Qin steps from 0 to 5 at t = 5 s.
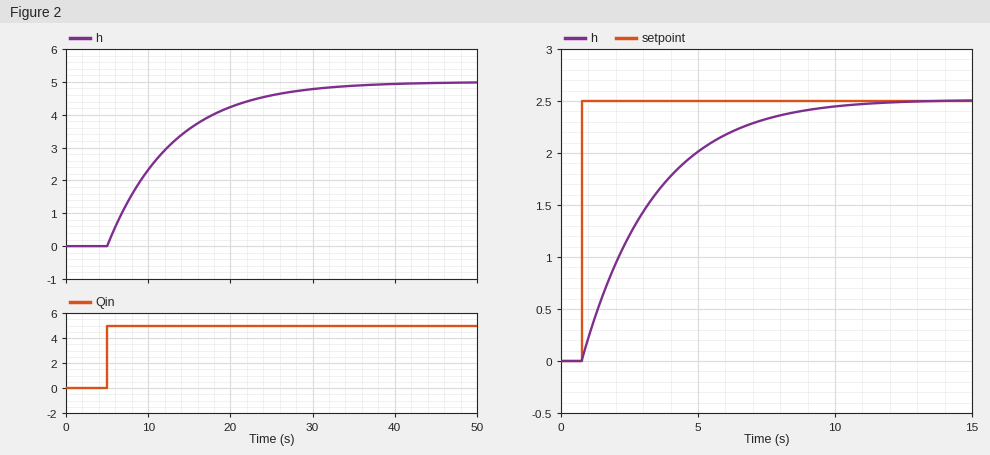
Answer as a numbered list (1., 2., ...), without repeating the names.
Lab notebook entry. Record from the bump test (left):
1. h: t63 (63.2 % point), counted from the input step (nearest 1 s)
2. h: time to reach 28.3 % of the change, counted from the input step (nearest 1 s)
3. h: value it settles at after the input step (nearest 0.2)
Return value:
1. 8 s
2. 3 s
3. 5.0
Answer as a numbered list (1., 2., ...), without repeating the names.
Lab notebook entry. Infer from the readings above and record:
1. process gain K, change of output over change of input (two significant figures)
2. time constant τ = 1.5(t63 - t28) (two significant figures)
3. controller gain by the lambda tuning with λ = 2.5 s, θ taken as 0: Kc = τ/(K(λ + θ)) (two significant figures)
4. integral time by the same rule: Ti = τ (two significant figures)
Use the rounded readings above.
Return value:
1. 1.0
2. 7.5 s
3. 3.0
4. 7.5 s
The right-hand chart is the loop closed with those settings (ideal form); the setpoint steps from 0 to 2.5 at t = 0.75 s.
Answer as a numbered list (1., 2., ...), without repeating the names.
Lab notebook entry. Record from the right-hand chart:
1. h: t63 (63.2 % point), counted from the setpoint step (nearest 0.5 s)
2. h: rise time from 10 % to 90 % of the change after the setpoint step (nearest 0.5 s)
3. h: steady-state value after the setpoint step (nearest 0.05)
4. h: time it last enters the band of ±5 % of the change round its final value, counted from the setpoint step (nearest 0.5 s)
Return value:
1. 2.5 s
2. 5.5 s
3. 2.50
4. 7.5 s
